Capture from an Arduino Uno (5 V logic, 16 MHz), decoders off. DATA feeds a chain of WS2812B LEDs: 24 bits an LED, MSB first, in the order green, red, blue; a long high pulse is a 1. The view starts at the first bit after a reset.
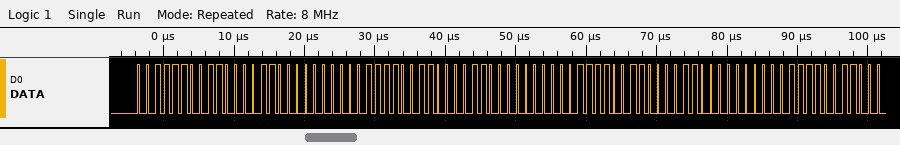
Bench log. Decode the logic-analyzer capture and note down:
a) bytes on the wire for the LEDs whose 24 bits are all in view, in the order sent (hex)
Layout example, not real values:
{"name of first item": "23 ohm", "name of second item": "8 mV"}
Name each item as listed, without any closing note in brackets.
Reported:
{"bytes on the wire for the LEDs whose 24 bits are all in view, in the order sent": "3C C3 00 3C C3 00 3C C3 00"}
